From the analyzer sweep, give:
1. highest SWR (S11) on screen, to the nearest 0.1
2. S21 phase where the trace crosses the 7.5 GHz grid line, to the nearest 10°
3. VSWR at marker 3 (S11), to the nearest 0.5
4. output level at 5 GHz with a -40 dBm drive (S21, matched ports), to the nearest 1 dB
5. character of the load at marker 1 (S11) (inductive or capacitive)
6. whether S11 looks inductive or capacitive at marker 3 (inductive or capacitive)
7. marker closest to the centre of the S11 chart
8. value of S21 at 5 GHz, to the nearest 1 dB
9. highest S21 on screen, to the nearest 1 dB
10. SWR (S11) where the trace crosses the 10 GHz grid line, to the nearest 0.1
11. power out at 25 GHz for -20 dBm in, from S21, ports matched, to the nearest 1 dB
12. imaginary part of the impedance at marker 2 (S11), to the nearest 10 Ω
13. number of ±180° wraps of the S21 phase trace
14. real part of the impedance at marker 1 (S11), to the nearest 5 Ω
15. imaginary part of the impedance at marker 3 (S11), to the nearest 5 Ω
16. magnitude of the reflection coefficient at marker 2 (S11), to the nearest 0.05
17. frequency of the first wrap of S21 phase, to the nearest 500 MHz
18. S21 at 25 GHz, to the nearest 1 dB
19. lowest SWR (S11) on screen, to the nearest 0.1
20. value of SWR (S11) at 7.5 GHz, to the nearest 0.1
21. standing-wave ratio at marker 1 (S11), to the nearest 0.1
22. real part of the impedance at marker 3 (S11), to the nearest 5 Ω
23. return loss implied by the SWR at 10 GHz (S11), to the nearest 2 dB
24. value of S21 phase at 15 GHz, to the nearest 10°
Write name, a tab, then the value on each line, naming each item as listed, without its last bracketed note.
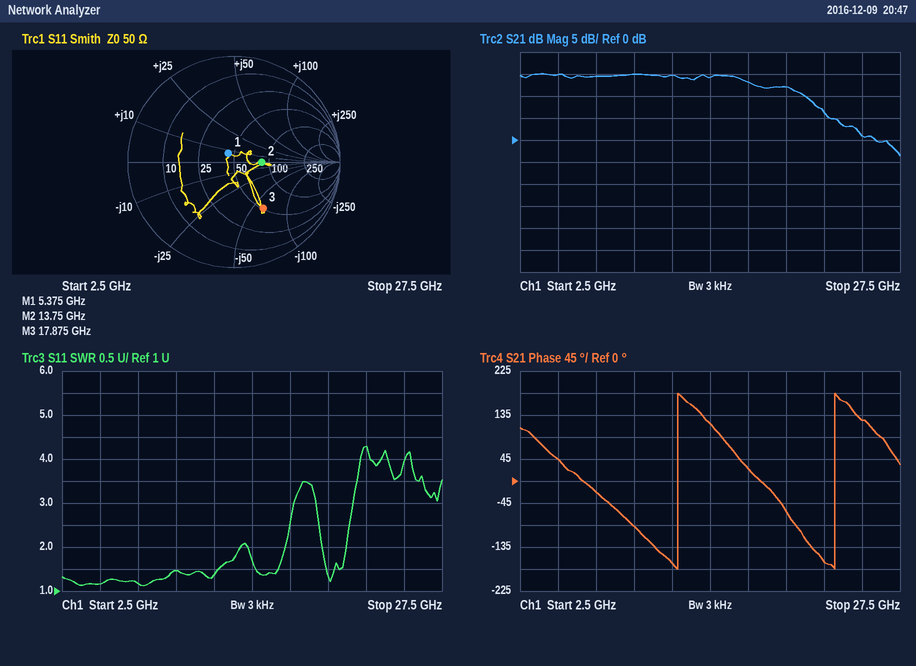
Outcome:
highest SWR (S11) on screen, to the nearest 0.1	4.3
S21 phase where the trace crosses the 7.5 GHz grid line, to the nearest 10°	-20°
VSWR at marker 3 (S11), to the nearest 0.5	3.0
output level at 5 GHz with a -40 dBm drive (S21, matched ports), to the nearest 1 dB	-25 dBm
character of the load at marker 1 (S11)	inductive
whether S11 looks inductive or capacitive at marker 3	capacitive
marker closest to the centre of the S11 chart	marker 1
value of S21 at 5 GHz, to the nearest 1 dB	15 dB
highest S21 on screen, to the nearest 1 dB	15 dB
SWR (S11) where the trace crosses the 10 GHz grid line, to the nearest 0.1	1.5
power out at 25 GHz for -20 dBm in, from S21, ports matched, to the nearest 1 dB	-19 dBm
imaginary part of the impedance at marker 2 (S11), to the nearest 10 Ω	0 Ω
number of ±180° wraps of the S21 phase trace	2
real part of the impedance at marker 1 (S11), to the nearest 5 Ω	45 Ω
imaginary part of the impedance at marker 3 (S11), to the nearest 5 Ω	-60 Ω
magnitude of the reflection coefficient at marker 2 (S11), to the nearest 0.05	0.25
frequency of the first wrap of S21 phase, to the nearest 500 MHz	13.0 GHz
S21 at 25 GHz, to the nearest 1 dB	1 dB
lowest SWR (S11) on screen, to the nearest 0.1	1.1
value of SWR (S11) at 7.5 GHz, to the nearest 0.1	1.2
standing-wave ratio at marker 1 (S11), to the nearest 0.1	1.2
real part of the impedance at marker 3 (S11), to the nearest 5 Ω	50 Ω
return loss implied by the SWR at 10 GHz (S11), to the nearest 2 dB	14 dB
value of S21 phase at 15 GHz, to the nearest 10°	120°
